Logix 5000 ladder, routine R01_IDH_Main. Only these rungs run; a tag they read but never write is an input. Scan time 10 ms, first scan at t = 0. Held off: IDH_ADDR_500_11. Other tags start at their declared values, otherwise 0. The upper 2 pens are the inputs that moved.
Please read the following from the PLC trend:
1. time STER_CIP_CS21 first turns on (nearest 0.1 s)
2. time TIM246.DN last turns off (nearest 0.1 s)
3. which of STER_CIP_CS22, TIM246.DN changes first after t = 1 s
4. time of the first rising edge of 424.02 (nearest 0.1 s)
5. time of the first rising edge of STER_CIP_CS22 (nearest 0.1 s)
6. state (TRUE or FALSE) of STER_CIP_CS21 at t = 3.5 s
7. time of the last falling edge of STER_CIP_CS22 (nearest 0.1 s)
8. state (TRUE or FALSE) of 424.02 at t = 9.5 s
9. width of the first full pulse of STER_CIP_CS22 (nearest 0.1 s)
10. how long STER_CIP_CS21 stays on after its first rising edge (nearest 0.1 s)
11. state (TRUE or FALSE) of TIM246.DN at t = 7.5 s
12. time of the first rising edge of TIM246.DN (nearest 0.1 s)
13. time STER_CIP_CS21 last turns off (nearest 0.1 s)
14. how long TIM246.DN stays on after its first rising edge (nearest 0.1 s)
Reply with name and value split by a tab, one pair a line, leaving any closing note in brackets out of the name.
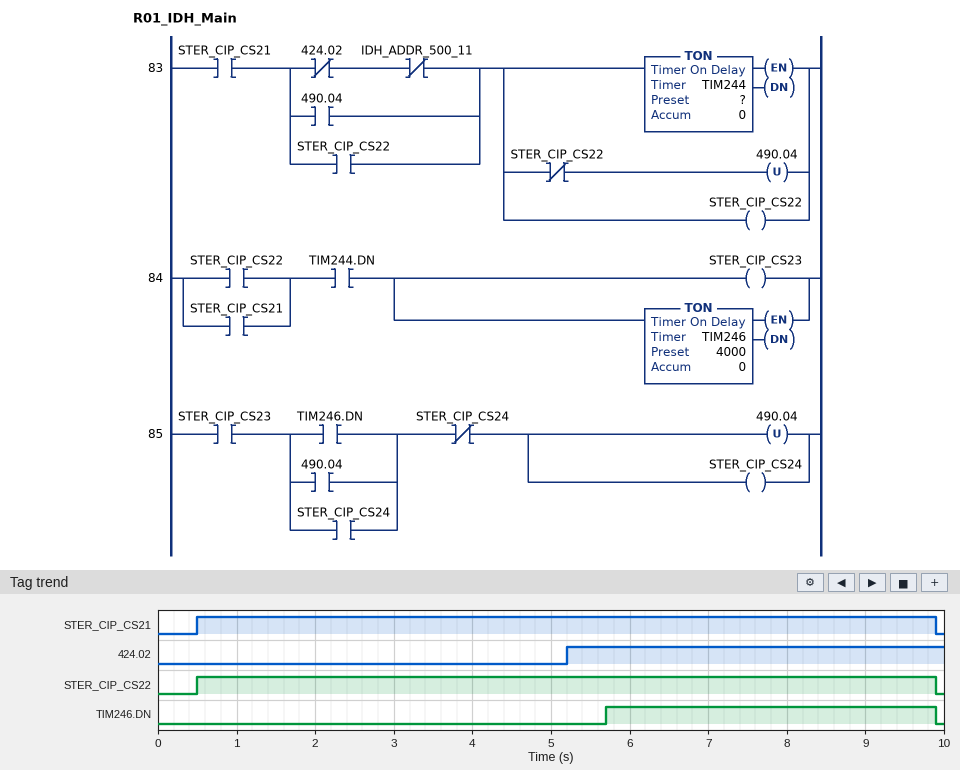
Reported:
time STER_CIP_CS21 first turns on	0.5 s
time TIM246.DN last turns off	9.9 s
which of STER_CIP_CS22, TIM246.DN changes first after t = 1 s	TIM246.DN
time of the first rising edge of 424.02	5.2 s
time of the first rising edge of STER_CIP_CS22	0.5 s
state (TRUE or FALSE) of STER_CIP_CS21 at t = 3.5 s	TRUE
time of the last falling edge of STER_CIP_CS22	9.9 s
state (TRUE or FALSE) of 424.02 at t = 9.5 s	TRUE
width of the first full pulse of STER_CIP_CS22	9.4 s
how long STER_CIP_CS21 stays on after its first rising edge	9.4 s
state (TRUE or FALSE) of TIM246.DN at t = 7.5 s	TRUE
time of the first rising edge of TIM246.DN	5.7 s
time STER_CIP_CS21 last turns off	9.9 s
how long TIM246.DN stays on after its first rising edge	4.2 s
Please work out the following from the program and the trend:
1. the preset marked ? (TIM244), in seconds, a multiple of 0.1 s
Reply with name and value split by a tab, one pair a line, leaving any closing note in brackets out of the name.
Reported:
the preset marked ? (TIM244), in seconds, a multiple of 0.1 s	1.2 s
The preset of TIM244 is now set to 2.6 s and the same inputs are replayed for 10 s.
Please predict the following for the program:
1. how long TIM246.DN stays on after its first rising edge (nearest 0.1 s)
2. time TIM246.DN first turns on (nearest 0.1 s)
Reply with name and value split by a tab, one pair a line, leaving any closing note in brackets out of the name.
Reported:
how long TIM246.DN stays on after its first rising edge	2.8 s
time TIM246.DN first turns on	7.1 s
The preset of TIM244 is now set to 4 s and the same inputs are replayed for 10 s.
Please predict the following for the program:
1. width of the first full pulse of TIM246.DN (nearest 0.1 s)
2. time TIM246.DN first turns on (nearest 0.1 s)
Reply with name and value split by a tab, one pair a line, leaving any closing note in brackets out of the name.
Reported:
width of the first full pulse of TIM246.DN	1.4 s
time TIM246.DN first turns on	8.5 s
